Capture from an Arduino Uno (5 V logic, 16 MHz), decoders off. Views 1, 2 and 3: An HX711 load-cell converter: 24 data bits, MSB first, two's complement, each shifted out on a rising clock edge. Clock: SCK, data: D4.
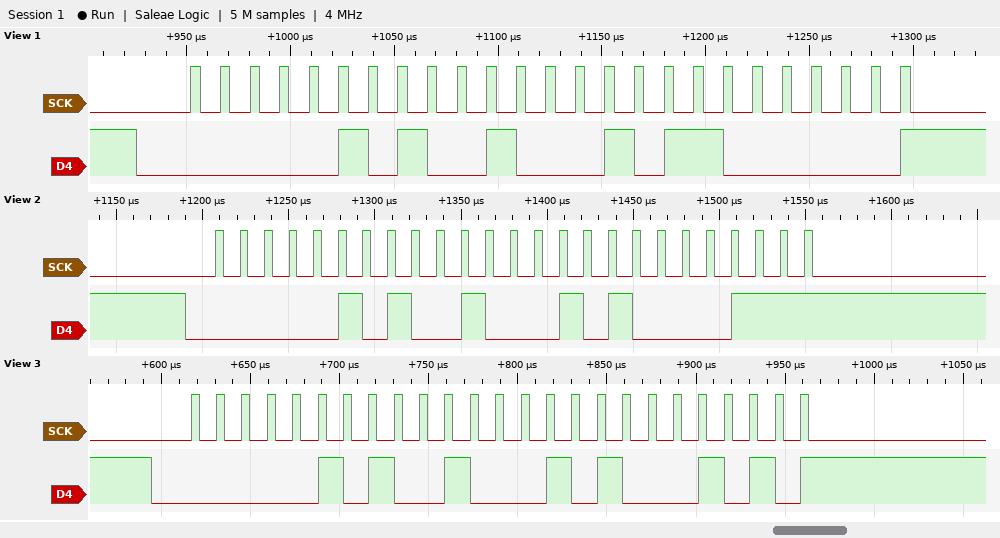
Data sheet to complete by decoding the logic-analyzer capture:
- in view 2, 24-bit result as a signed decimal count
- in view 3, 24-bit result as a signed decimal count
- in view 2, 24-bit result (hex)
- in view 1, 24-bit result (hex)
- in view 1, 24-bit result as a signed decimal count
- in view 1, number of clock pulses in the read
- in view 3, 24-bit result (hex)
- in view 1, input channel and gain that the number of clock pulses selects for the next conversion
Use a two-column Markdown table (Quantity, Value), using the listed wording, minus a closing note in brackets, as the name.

| Quantity | Value |
|---|---|
| in view 2, 24-bit result as a signed decimal count | 336519 |
| in view 3, 24-bit result as a signed decimal count | 336522 |
| in view 2, 24-bit result | 0x052287 |
| in view 1, 24-bit result | 0x0522C0 |
| in view 1, 24-bit result as a signed decimal count | 336576 |
| in view 1, number of clock pulses in the read | 25 |
| in view 3, 24-bit result | 0x05228A |
| in view 1, input channel and gain that the number of clock pulses selects for the next conversion | channel A, gain 128 |
